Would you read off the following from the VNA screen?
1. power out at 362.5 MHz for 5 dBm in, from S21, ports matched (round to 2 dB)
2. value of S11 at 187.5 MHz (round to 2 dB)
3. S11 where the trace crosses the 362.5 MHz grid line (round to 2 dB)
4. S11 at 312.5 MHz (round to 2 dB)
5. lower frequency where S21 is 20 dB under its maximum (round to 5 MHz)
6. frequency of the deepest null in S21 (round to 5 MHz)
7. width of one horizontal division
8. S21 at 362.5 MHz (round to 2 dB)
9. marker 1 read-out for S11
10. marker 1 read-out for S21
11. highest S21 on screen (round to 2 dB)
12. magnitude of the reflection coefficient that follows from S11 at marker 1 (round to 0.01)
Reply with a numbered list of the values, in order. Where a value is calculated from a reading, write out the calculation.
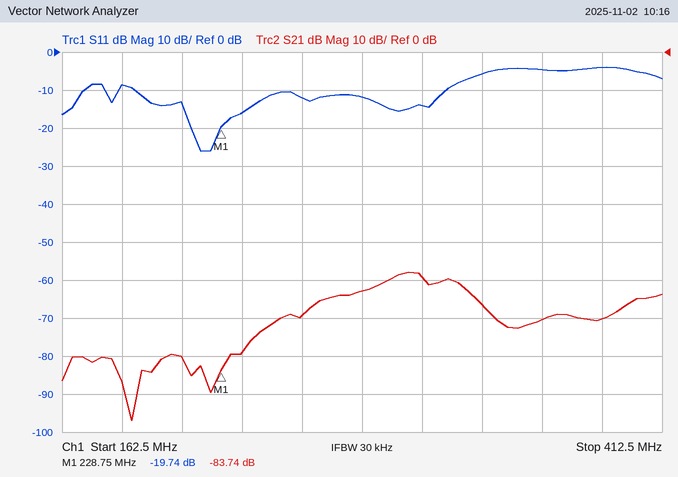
1. 5 dBm + (-70 dB) = -66 dBm
2. -8 dB
3. -4 dB
4. -14 dB
5. 240 MHz
6. 190 MHz
7. 25 MHz
8. -70 dB
9. -19.74 dB
10. -83.74 dB
11. -58 dB
12. 10^(-19.74/20) ≈ 0.10
